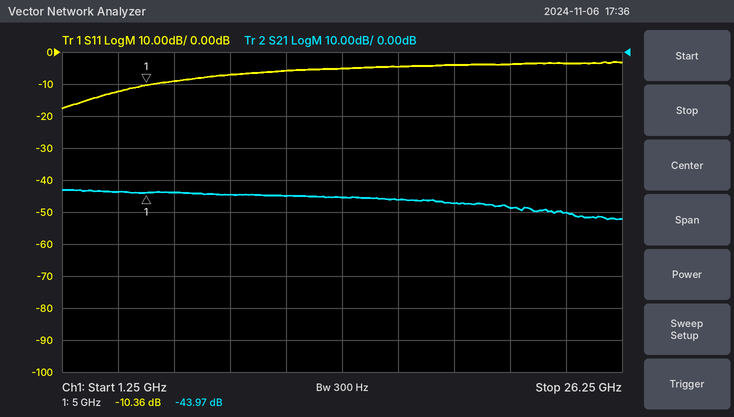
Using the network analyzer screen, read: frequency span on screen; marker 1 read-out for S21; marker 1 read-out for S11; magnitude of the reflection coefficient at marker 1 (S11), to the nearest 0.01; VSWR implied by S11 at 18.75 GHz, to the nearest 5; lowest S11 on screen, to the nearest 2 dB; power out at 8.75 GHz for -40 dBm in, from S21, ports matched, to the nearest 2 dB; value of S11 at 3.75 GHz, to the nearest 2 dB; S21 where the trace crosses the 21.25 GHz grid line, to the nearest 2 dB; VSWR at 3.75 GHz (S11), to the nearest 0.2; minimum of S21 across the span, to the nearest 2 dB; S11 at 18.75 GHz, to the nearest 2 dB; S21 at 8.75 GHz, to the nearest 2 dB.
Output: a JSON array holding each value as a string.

["25 GHz", "-43.97 dB", "-10.36 dB", "0.30", "5", "-18 dB", "-84 dBm", "-12 dB", "-48 dB", "1.6", "-52 dB", "-4 dB", "-44 dB"]
